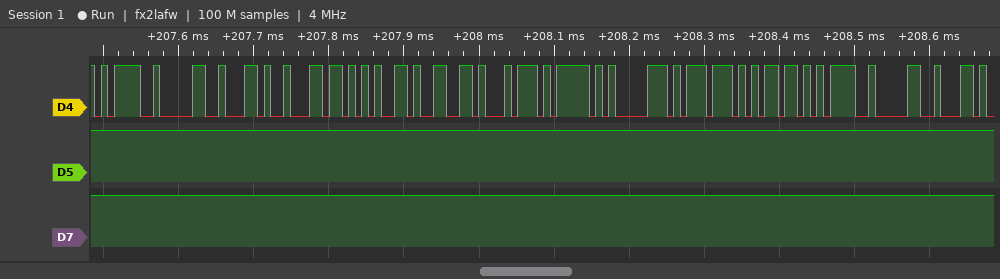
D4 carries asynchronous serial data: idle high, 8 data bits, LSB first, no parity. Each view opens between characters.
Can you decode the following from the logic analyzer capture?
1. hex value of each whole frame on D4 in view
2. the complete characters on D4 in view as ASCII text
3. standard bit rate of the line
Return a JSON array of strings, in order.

["3D, 30, 2C, 6C, 65, 66, 74, 5F, 70, 77, 6D, 3D, 30", "\"=0,left_pwm=0\"", "115200 baud"]
